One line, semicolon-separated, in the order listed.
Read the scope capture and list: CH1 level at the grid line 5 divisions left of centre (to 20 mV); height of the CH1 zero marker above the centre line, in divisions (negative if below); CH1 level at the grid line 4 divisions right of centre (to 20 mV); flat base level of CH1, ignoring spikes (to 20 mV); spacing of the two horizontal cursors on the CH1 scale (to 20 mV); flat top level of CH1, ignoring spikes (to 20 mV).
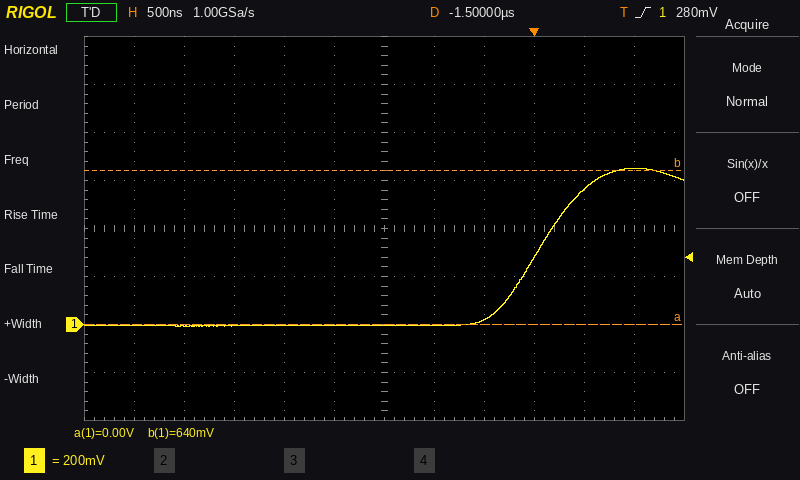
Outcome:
0 mV; -2.0 div; 560 mV; 0 mV; 640 mV; 640 mV
